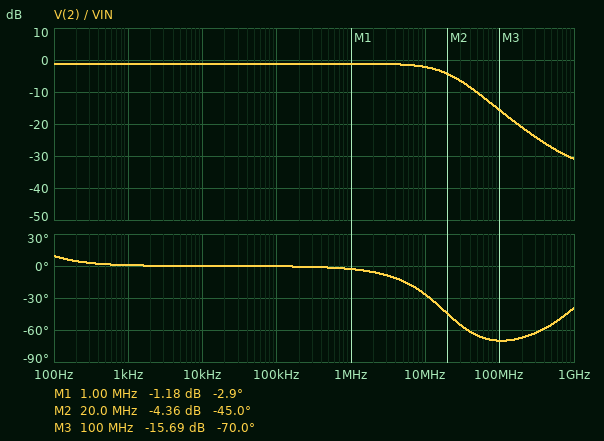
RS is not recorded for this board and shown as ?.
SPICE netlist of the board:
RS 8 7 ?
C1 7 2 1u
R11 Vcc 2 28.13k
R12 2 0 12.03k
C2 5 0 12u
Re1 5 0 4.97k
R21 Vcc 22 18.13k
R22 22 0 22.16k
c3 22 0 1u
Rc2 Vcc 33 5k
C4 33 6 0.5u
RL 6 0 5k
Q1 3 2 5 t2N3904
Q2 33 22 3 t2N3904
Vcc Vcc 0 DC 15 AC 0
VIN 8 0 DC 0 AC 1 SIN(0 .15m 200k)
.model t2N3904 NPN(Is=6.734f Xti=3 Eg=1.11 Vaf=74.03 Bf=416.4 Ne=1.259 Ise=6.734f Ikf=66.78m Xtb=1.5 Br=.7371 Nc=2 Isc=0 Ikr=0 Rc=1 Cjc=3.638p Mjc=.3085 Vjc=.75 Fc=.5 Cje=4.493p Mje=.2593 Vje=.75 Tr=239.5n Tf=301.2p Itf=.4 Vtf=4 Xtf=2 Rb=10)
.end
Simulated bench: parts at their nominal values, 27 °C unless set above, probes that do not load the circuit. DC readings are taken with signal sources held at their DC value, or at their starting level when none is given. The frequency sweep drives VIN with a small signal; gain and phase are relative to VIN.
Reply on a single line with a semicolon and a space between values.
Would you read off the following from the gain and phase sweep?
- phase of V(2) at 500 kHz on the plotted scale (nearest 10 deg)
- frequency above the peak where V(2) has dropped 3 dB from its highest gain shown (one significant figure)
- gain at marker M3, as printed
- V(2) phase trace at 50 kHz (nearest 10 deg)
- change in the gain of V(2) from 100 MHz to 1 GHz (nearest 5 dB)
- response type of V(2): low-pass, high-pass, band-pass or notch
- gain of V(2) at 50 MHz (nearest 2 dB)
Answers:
0 deg; 20 MHz; -15.69 dB; 0 deg; -15 dB; low-pass; -10 dB
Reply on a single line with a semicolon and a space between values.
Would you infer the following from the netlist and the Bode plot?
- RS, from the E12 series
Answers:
470 Ω
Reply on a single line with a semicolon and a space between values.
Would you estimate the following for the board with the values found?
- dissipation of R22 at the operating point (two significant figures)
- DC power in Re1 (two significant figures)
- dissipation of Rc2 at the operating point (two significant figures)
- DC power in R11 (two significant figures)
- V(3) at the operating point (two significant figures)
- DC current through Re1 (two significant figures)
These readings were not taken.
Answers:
3.0 mW; 2.9 mW; 2.8 mW; 4.0 mW; 7.5 V; 760 µA
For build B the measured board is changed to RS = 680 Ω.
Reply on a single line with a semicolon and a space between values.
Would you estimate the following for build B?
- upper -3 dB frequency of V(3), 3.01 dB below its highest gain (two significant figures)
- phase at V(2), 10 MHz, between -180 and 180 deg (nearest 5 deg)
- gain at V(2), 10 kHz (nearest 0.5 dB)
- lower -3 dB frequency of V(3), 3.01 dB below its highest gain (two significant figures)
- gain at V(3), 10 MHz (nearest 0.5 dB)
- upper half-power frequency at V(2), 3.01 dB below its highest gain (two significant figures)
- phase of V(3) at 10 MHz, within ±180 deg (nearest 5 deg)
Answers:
16 MHz; -35 deg; -1.5 dB; 370 Hz; -3.0 dB; 13 MHz; 145 deg
